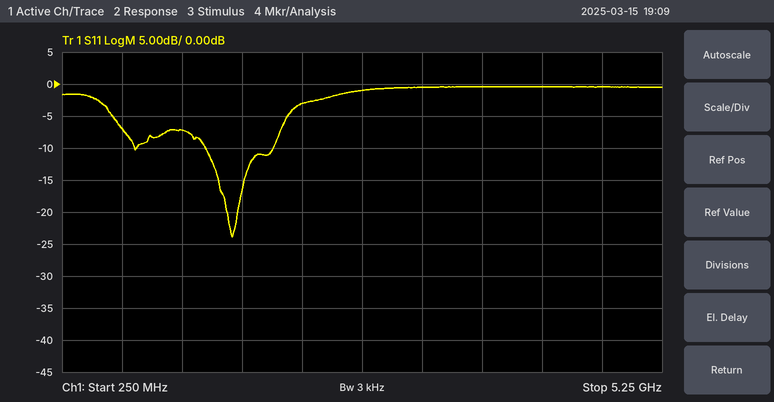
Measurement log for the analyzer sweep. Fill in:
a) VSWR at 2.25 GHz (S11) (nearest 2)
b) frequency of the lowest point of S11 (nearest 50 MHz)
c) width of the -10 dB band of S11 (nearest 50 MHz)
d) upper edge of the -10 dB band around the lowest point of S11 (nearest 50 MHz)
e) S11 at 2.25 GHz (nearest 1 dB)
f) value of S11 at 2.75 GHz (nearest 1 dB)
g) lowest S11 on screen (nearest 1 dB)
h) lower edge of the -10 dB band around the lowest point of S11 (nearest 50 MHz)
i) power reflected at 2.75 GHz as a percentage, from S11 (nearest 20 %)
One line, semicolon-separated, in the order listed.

6; 1.65 GHz; 550 MHz; 2.00 GHz; -3 dB; -1 dB; -24 dB; 1.45 GHz; 80 %
